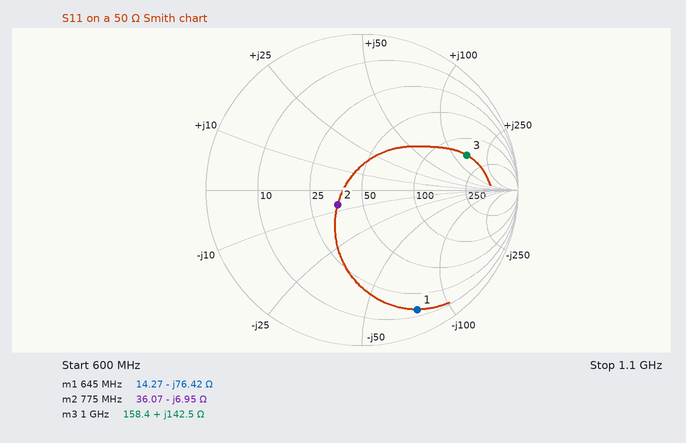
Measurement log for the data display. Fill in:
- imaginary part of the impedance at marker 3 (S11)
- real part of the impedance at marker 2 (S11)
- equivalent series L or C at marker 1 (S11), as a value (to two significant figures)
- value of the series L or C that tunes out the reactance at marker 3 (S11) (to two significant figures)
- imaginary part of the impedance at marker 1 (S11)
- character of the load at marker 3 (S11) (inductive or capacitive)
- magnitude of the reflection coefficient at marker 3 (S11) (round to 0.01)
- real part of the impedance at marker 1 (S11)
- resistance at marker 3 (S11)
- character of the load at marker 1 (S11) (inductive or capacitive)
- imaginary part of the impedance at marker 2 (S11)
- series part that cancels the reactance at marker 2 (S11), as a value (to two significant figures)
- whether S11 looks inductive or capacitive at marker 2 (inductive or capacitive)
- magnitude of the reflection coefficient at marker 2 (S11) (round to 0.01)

+142.5 Ω
36.07 Ω
3.2 pF
1.1 pF
-76.42 Ω
inductive
0.71
14.27 Ω
158.4 Ω
capacitive
-6.95 Ω
1.4 nH
capacitive
0.18
